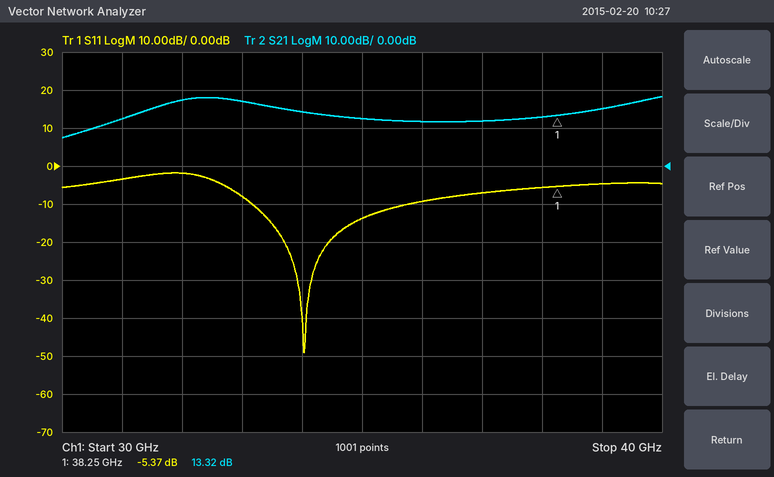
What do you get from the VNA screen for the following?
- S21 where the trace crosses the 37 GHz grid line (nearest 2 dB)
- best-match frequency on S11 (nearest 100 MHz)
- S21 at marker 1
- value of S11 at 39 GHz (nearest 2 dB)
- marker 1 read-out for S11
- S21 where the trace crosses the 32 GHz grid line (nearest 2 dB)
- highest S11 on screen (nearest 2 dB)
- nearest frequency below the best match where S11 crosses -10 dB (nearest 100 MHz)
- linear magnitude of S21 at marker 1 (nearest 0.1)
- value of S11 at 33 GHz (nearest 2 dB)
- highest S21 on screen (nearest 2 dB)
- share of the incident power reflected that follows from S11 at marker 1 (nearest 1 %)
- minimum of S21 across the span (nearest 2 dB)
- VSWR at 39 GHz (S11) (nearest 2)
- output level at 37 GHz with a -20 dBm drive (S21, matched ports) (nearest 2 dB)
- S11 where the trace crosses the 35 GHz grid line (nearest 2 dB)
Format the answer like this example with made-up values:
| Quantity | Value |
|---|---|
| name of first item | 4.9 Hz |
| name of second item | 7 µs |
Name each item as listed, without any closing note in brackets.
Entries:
| Quantity | Value |
|---|---|
| S21 where the trace crosses the 37 GHz grid line | 12 dB |
| best-match frequency on S11 | 34.0 GHz |
| S21 at marker 1 | 13.32 dB |
| value of S11 at 39 GHz | -4 dB |
| marker 1 read-out for S11 | -5.37 dB |
| S21 where the trace crosses the 32 GHz grid line | 18 dB |
| highest S11 on screen | -2 dB |
| nearest frequency below the best match where S11 crosses -10 dB | 33.2 GHz |
| linear magnitude of S21 at marker 1 | 4.6 |
| value of S11 at 33 GHz | -8 dB |
| highest S21 on screen | 18 dB |
| share of the incident power reflected that follows from S11 at marker 1 | 29 % |
| minimum of S21 across the span | 8 dB |
| VSWR at 39 GHz (S11) | 4 |
| output level at 37 GHz with a -20 dBm drive (S21, matched ports) | -8 dBm |
| S11 where the trace crosses the 35 GHz grid line | -14 dB |
